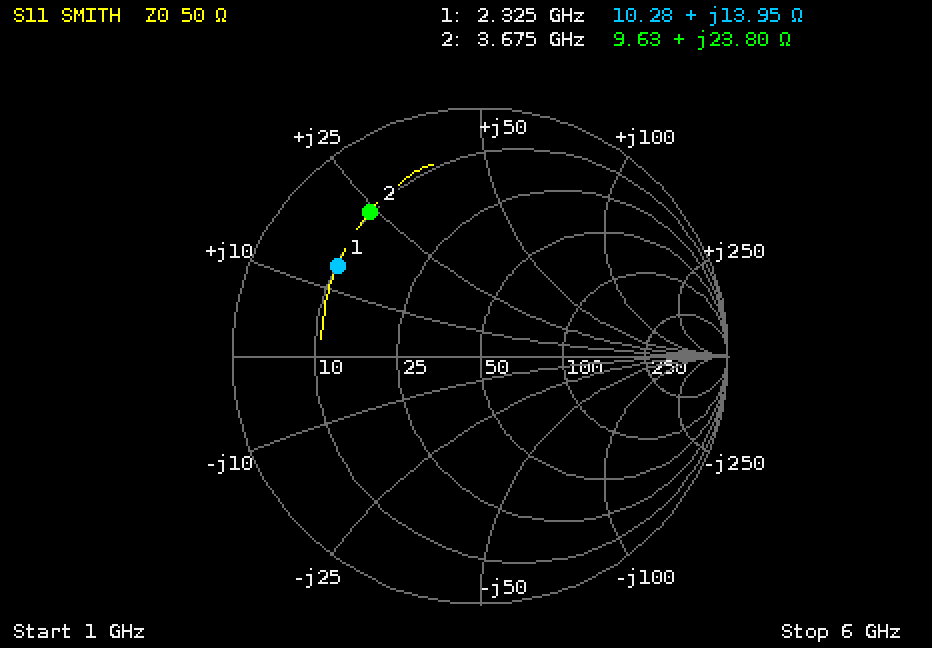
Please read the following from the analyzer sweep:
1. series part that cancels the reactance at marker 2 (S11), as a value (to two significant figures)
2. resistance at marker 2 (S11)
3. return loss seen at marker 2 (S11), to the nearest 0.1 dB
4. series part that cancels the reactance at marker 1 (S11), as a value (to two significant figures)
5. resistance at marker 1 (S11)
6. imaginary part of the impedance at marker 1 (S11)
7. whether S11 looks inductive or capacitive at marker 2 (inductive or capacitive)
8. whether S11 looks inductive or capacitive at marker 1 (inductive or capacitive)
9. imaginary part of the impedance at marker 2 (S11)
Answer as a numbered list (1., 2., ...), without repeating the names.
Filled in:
1. 1.8 pF
2. 9.63 Ω
3. 2.7 dB
4. 4.9 pF
5. 10.28 Ω
6. +13.95 Ω
7. inductive
8. inductive
9. +23.80 Ω
